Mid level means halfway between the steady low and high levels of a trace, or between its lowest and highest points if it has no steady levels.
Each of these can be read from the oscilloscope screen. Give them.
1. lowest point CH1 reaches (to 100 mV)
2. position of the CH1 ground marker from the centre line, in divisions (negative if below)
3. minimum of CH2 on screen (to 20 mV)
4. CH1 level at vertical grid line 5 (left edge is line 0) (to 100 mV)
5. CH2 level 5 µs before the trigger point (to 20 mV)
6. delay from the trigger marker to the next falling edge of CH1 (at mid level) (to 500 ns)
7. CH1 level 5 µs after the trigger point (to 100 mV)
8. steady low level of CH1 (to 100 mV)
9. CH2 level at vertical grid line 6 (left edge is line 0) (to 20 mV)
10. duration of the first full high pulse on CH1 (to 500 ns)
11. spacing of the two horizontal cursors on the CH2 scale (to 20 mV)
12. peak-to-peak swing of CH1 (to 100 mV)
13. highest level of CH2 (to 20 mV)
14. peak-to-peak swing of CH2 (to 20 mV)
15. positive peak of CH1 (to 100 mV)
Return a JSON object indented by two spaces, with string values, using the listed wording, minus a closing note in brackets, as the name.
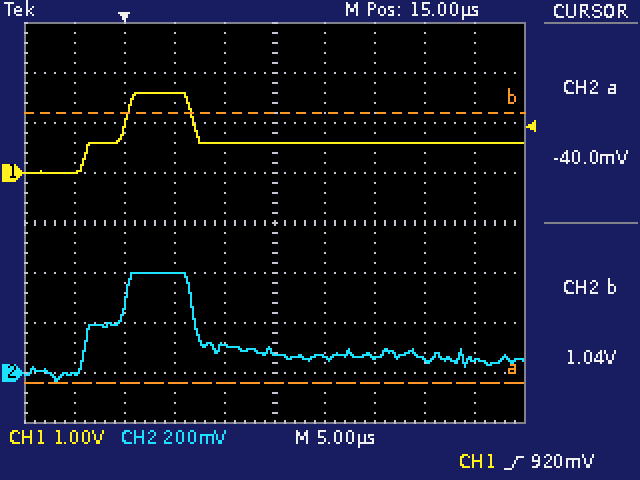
{
  "lowest point CH1 reaches": "0.0 V",
  "position of the CH1 ground marker from the centre line, in divisions": "+1.0 div",
  "minimum of CH2 on screen": "-40 mV",
  "CH1 level at vertical grid line 5 (left edge is line 0)": "600 mV",
  "CH2 level 5 µs before the trigger point": "0 mV",
  "delay from the trigger marker to the next falling edge of CH1 (at mid level)": "7.0 µs",
  "CH1 level 5 µs after the trigger point": "1.6 V",
  "steady low level of CH1": "600 mV",
  "CH2 level at vertical grid line 6 (left edge is line 0)": "60 mV",
  "duration of the first full high pulse on CH1": "6.5 µs",
  "spacing of the two horizontal cursors on the CH2 scale": "1.08 V",
  "peak-to-peak swing of CH1": "1.6 V",
  "highest level of CH2": "400 mV",
  "peak-to-peak swing of CH2": "440 mV",
  "positive peak of CH1": "1.6 V"
}
